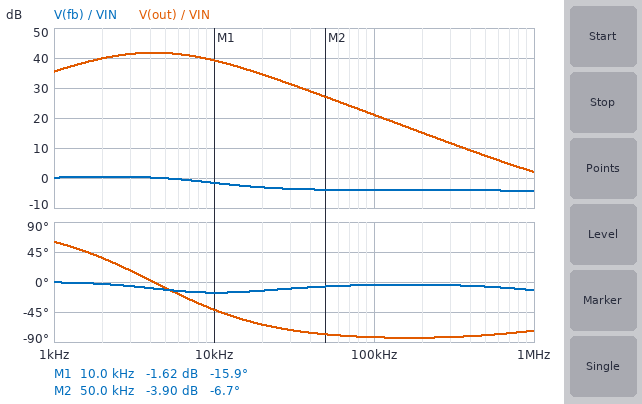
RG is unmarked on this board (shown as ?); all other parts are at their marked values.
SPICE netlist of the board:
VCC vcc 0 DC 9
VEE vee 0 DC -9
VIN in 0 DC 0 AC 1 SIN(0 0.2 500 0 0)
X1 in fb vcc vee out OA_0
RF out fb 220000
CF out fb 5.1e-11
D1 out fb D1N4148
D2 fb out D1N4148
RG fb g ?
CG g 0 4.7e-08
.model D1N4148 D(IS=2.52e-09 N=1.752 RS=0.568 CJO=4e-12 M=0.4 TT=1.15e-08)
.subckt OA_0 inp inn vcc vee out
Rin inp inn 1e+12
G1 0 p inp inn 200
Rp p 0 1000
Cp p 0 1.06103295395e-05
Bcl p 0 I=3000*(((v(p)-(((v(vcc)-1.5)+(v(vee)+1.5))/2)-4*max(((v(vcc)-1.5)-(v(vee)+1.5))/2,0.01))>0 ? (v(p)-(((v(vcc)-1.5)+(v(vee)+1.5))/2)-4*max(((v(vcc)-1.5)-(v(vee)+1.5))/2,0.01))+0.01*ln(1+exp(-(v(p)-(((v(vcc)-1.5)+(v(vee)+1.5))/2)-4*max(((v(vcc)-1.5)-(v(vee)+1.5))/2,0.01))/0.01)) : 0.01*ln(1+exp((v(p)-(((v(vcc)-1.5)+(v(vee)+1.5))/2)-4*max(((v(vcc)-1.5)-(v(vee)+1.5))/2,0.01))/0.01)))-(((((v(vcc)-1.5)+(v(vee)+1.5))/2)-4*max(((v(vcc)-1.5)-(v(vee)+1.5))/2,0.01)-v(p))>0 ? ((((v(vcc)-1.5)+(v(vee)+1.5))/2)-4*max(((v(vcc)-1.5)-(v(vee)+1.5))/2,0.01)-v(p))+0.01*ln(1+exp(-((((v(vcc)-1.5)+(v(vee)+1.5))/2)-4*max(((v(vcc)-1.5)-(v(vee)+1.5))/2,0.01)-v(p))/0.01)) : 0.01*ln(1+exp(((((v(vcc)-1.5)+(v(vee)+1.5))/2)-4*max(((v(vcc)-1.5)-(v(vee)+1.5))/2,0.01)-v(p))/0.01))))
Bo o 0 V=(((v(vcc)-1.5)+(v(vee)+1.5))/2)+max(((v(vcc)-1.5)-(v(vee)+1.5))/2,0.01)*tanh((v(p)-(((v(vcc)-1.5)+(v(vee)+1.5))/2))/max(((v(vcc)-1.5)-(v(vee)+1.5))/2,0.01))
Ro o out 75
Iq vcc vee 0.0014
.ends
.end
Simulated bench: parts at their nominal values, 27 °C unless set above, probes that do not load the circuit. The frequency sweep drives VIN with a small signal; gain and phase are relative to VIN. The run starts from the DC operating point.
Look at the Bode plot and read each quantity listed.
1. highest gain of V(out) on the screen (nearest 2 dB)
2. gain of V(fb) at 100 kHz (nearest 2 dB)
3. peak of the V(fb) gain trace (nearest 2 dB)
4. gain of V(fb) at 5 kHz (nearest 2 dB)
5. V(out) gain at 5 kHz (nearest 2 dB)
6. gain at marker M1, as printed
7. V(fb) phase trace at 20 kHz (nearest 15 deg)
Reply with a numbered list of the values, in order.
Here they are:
1. 42 dB
2. -4 dB
3. 0 dB
4. 0 dB
5. 42 dB
6. -1.62 dB
7. -15 deg
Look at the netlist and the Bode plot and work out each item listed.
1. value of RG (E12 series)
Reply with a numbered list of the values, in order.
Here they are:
1. 1.5 kΩ
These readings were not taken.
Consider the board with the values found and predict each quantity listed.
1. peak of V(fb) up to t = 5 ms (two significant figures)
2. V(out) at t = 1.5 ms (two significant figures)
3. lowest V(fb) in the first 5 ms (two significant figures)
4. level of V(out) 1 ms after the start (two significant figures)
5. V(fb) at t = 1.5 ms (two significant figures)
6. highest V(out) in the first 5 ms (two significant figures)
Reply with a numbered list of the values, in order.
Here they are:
1. 200 mV
2. -540 mV
3. -200 mV
4. -420 mV
5. -200 mV
6. 580 mV
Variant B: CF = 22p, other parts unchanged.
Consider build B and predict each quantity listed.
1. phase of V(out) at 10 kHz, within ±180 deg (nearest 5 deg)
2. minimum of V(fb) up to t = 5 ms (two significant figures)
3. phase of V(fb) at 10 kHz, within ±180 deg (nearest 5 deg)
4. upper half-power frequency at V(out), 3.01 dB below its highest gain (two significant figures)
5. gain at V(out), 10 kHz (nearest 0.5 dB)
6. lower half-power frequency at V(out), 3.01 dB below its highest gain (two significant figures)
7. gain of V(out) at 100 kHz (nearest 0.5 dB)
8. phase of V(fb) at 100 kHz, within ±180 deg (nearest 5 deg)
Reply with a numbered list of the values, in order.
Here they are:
1. -30 deg
2. -200 mV
3. -20 deg
4. 14 kHz
5. 41.0 dB
6. 1.8 kHz
7. 24.0 dB
8. -10 deg
